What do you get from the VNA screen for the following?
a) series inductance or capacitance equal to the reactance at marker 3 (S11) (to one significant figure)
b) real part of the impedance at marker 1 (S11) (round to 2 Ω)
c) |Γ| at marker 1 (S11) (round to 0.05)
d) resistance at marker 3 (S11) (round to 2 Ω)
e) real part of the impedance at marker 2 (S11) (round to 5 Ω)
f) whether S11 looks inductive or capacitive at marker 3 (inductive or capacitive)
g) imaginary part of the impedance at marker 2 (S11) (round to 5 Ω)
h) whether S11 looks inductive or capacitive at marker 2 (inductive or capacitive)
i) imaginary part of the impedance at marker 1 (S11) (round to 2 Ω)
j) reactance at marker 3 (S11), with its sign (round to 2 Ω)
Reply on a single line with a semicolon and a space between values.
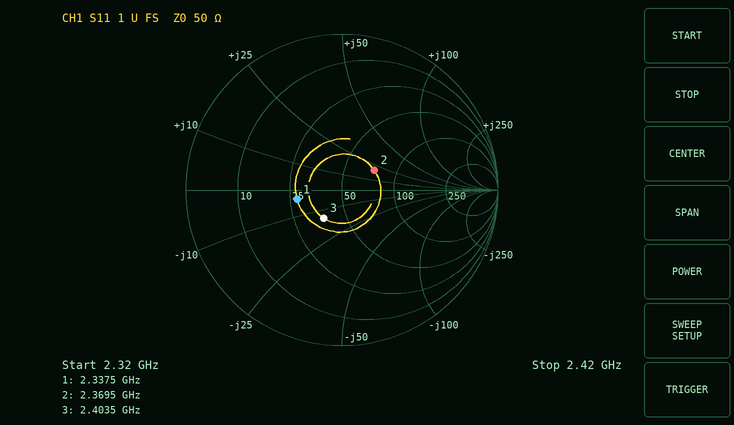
5 pF; 28 Ω; 0.30; 38 Ω; 75 Ω; capacitive; +20 Ω; inductive; -4 Ω; -14 Ω
